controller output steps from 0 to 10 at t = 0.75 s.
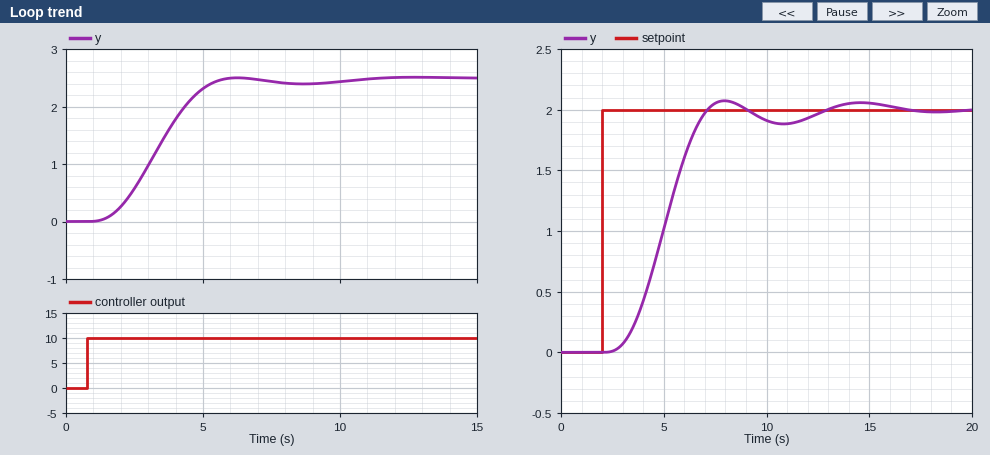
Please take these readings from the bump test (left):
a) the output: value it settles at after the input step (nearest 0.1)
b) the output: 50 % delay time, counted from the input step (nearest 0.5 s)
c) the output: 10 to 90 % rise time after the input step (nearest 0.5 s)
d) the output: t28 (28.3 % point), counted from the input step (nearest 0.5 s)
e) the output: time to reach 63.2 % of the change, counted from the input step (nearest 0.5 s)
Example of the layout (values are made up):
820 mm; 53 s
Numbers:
2.5; 2.5 s; 3.0 s; 2.0 s; 3.0 s
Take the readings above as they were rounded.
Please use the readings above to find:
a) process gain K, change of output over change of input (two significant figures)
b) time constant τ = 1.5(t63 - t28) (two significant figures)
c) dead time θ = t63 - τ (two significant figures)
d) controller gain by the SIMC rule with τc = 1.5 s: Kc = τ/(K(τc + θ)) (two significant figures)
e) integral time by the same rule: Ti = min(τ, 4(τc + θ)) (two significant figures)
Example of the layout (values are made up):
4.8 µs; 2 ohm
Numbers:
0.25; 1.5 s; 1.5 s; 2.0; 1.5 s
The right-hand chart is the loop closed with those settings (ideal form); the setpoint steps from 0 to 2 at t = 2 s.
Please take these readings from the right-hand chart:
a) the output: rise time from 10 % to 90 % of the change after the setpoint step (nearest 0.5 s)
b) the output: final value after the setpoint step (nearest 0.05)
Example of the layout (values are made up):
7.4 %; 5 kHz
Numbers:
3.0 s; 2.00
